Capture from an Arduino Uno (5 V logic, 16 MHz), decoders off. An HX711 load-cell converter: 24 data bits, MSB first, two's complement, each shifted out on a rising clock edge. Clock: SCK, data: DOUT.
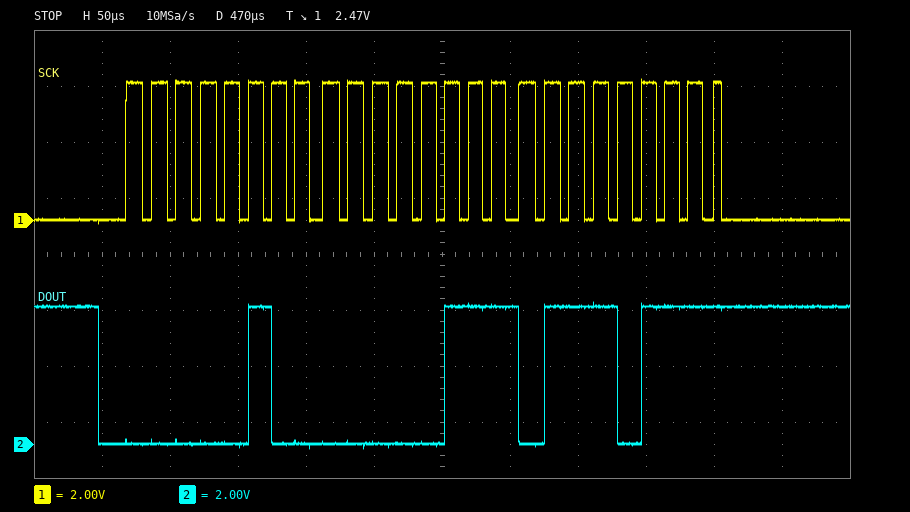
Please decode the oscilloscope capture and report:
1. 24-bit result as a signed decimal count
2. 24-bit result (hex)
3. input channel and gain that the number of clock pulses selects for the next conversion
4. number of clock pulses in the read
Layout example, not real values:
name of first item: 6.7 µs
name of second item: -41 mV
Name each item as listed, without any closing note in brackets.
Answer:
24-bit result as a signed decimal count: 264055
24-bit result: 0x040777
input channel and gain that the number of clock pulses selects for the next conversion: channel A, gain 128
number of clock pulses in the read: 25
